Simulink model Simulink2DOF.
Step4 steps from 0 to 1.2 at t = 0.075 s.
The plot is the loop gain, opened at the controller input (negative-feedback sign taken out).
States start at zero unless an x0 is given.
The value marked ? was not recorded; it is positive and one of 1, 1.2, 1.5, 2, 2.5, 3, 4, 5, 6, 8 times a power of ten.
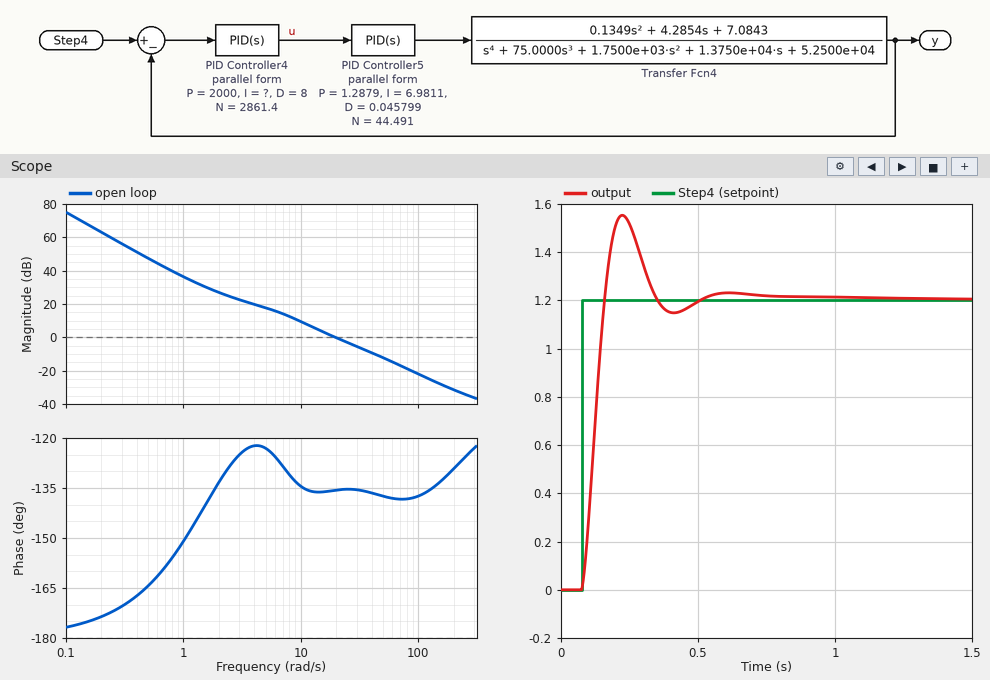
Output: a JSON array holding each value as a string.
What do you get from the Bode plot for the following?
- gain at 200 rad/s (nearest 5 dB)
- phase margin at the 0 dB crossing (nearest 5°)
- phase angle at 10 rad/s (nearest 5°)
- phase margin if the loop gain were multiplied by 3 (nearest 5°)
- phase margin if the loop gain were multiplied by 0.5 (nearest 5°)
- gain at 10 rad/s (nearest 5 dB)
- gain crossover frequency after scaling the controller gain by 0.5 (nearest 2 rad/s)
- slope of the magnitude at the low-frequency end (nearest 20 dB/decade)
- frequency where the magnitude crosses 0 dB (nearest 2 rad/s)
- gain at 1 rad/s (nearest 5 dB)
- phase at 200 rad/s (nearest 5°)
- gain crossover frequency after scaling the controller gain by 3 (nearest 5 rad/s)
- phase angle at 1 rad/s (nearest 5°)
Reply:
["-30 dB", "45°", "-135°", "45°", "45°", "10 dB", "12 rad/s", "-40 dB/decade", "20 rad/s", "35 dB", "-130°", "40 rad/s", "-150°"]
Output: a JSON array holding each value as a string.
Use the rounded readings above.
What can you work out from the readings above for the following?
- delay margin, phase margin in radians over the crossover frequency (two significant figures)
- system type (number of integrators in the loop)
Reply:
["0.039 s", "2"]
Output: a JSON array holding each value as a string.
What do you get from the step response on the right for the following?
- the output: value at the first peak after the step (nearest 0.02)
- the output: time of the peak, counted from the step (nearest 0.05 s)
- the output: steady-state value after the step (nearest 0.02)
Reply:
["1.56", "0.15 s", "1.20"]
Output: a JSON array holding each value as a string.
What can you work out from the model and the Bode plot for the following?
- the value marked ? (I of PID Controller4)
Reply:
["60000"]
